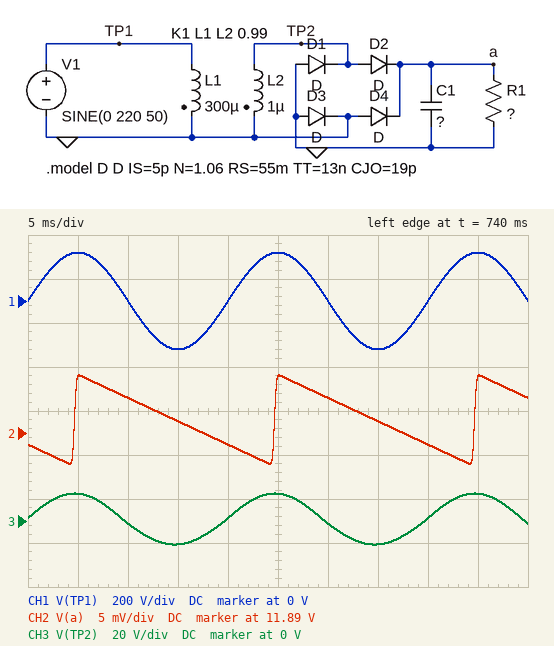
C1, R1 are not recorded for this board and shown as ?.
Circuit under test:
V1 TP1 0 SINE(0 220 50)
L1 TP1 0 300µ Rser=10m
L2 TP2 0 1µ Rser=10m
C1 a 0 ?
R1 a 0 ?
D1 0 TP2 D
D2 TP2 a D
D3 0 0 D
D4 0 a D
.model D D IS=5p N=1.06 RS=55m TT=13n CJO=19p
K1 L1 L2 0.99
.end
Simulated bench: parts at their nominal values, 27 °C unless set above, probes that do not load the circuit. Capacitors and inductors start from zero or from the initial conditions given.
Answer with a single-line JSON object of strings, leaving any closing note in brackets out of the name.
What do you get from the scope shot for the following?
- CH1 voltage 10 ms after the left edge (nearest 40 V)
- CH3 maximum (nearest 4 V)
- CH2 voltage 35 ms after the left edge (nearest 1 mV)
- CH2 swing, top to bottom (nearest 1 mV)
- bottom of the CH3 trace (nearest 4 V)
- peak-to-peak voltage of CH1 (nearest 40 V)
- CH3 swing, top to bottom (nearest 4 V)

{"CH1 voltage 10 ms after the left edge": "0 V", "CH3 maximum": "12 V", "CH2 voltage 35 ms after the left edge": "11.896 V", "CH2 swing, top to bottom": "10 mV", "bottom of the CH3 trace": "-12 V", "peak-to-peak voltage of CH1": "440 V", "CH3 swing, top to bottom": "24 V"}
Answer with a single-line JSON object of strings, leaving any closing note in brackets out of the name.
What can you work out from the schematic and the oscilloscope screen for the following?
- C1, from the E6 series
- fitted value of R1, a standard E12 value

{"C1, from the E6 series": "680 µF", "fitted value of R1, a standard E12 value": "33 kΩ"}
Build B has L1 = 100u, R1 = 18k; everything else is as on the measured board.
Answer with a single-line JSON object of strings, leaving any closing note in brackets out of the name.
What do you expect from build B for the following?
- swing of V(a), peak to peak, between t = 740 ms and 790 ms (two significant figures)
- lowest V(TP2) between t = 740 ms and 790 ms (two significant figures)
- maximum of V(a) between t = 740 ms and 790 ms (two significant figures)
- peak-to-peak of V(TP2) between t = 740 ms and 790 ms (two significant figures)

{"swing of V(a), peak to peak, between t = 740 ms and 790 ms": "32 mV", "lowest V(TP2) between t = 740 ms and 790 ms": "-18 V", "maximum of V(a) between t = 740 ms and 790 ms": "20 V", "peak-to-peak of V(TP2) between t = 740 ms and 790 ms": "38 V"}
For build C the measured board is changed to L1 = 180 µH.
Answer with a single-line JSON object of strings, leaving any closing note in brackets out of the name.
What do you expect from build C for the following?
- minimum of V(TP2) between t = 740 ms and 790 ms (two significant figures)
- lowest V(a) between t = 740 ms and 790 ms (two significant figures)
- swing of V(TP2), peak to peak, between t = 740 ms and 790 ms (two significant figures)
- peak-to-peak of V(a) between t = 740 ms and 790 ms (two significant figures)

{"minimum of V(TP2) between t = 740 ms and 790 ms": "-14 V", "lowest V(a) between t = 740 ms and 790 ms": "15 V", "swing of V(TP2), peak to peak, between t = 740 ms and 790 ms": "30 V", "peak-to-peak of V(a) between t = 740 ms and 790 ms": "13 mV"}
